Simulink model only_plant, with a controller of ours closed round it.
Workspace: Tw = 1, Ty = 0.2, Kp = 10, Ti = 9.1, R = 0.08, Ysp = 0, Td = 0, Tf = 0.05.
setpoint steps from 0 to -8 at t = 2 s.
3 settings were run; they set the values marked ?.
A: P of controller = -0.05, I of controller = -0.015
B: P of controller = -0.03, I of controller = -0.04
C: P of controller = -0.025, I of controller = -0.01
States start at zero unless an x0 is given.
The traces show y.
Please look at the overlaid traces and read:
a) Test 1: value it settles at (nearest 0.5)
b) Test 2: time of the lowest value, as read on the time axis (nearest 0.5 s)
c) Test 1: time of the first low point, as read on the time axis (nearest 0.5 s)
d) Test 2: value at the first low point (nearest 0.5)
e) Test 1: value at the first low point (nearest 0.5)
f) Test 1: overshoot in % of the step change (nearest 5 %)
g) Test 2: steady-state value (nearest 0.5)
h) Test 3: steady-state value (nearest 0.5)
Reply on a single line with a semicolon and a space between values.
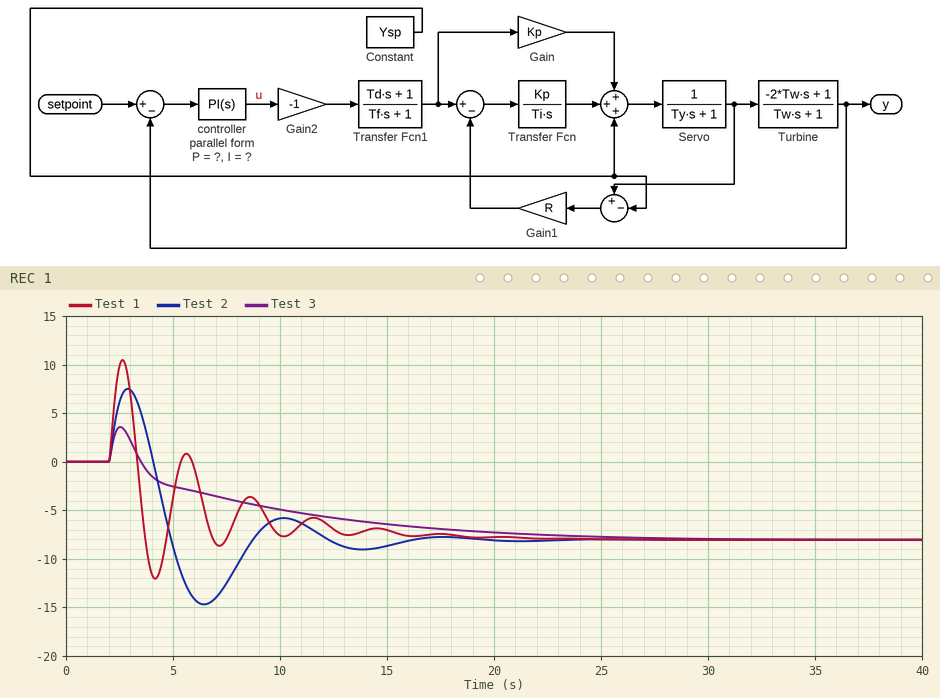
-8.0; 6.5 s; 4.0 s; -14.5; -12.0; 50 %; -8.0; -8.0
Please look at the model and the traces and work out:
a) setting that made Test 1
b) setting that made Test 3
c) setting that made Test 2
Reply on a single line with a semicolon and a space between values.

A; C; B
